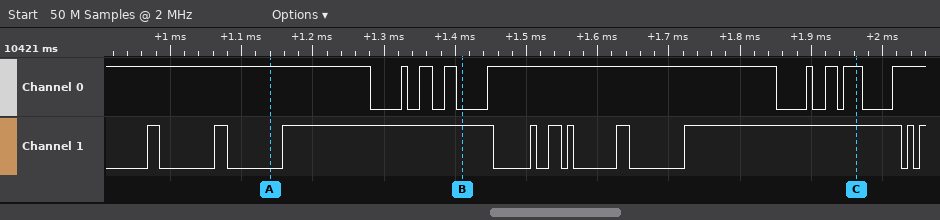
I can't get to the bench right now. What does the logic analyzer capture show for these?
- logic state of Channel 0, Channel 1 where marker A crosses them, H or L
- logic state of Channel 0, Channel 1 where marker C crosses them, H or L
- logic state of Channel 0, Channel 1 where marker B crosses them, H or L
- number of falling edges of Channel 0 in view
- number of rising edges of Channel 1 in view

Channel 0=H, Channel 1=L
Channel 0=H, Channel 1=H
Channel 0=L, Channel 1=H
8
10
